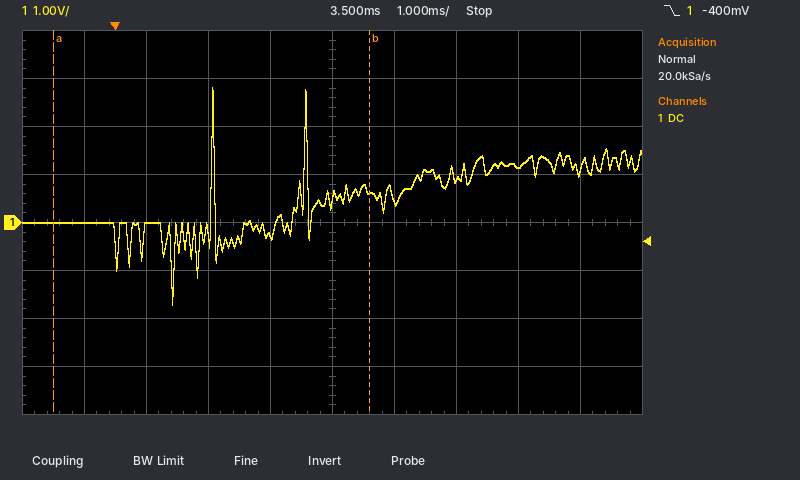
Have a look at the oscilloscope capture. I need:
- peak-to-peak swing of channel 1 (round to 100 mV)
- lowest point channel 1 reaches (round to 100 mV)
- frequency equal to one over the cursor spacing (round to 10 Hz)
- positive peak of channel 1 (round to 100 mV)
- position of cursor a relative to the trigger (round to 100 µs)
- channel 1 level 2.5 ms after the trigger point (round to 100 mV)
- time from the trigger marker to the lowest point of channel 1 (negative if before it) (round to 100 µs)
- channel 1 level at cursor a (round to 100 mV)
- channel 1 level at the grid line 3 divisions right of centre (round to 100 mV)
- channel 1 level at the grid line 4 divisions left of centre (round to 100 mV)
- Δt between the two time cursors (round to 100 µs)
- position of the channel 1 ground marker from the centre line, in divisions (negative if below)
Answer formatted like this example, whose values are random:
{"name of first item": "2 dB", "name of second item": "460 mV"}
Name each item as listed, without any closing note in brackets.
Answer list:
{"peak-to-peak swing of channel 1": "4.5 V", "lowest point channel 1 reaches": "-1.7 V", "frequency equal to one over the cursor spacing": "200 Hz", "positive peak of channel 1": "2.8 V", "position of cursor a relative to the trigger": "-1.0 ms", "channel 1 level 2.5 ms after the trigger point": "-300 mV", "time from the trigger marker to the lowest point of channel 1 (negative if before it)": "+900 µs", "channel 1 level at cursor a": "0.0 V", "channel 1 level at the grid line 3 divisions right of centre": "1.2 V", "channel 1 level at the grid line 4 divisions left of centre": "0.0 V", "Δt between the two time cursors": "5.1 ms", "position of the channel 1 ground marker from the centre line, in divisions": "0.0 div"}
